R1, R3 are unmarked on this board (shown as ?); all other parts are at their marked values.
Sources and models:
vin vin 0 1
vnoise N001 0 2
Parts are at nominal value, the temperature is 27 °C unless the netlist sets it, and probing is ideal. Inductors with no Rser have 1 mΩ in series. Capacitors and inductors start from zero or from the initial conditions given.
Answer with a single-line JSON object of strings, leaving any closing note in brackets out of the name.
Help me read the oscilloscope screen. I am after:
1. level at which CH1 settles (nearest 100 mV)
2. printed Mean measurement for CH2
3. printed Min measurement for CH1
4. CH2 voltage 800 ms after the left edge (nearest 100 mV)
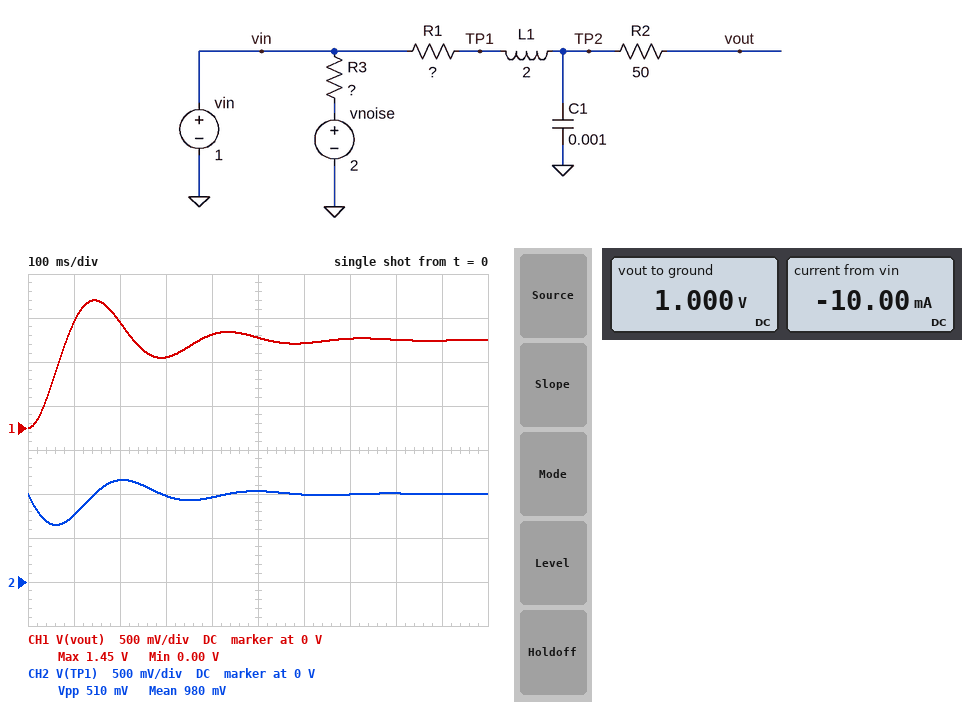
{"level at which CH1 settles": "1.0 V", "printed Mean measurement for CH2": "980 mV", "printed Min measurement for CH1": "0.00 V", "CH2 voltage 800 ms after the left edge": "1.0 V"}
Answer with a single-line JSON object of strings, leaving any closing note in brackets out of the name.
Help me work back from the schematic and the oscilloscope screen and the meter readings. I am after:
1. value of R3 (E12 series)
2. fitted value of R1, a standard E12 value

{"value of R3": "100 Ω", "fitted value of R1, a standard E12 value": "22 Ω"}
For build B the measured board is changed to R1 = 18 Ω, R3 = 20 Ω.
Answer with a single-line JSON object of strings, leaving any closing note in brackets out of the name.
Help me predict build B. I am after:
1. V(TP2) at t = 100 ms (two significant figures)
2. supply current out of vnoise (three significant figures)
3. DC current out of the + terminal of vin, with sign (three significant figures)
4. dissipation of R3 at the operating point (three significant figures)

{"V(TP2) at t = 100 ms": "1.3 V", "supply current out of vnoise": "50.0 mA", "DC current out of the + terminal of vin, with sign": "-50.0 mA", "dissipation of R3 at the operating point": "50.0 mW"}
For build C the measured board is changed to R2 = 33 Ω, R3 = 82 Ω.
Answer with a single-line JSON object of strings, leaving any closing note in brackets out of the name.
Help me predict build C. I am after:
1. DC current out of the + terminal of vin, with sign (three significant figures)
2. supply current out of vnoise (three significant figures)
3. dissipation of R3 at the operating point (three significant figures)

{"DC current out of the + terminal of vin, with sign": "-12.2 mA", "supply current out of vnoise": "12.2 mA", "dissipation of R3 at the operating point": "12.2 mW"}
